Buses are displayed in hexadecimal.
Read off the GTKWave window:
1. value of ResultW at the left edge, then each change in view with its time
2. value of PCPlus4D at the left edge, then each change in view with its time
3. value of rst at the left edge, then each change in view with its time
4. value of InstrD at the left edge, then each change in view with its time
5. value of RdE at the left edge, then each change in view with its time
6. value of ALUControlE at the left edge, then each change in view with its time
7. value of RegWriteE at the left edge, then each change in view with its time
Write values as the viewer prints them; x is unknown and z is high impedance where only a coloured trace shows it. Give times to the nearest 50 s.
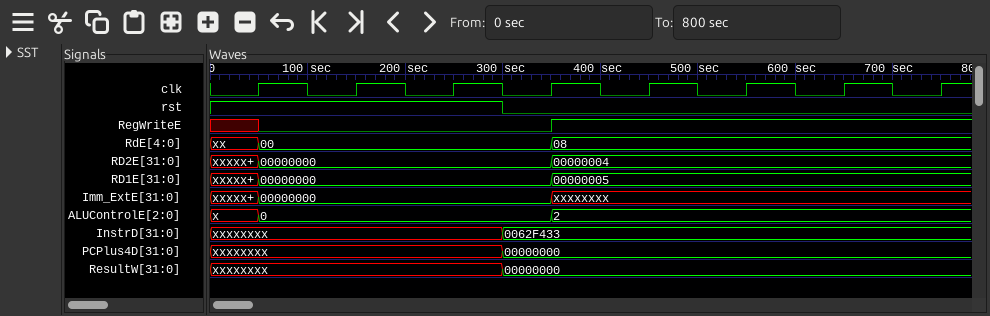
xxxxxxxx, 00000000 at 300 s
xxxxxxxx, 00000000 at 300 s
1, 0 at 300 s
xxxxxxxx, 0062F433 at 300 s
xx, 00 at 50 s, 08 at 350 s
x, 0 at 50 s, 2 at 350 s
x, 0 at 50 s, 1 at 350 s
